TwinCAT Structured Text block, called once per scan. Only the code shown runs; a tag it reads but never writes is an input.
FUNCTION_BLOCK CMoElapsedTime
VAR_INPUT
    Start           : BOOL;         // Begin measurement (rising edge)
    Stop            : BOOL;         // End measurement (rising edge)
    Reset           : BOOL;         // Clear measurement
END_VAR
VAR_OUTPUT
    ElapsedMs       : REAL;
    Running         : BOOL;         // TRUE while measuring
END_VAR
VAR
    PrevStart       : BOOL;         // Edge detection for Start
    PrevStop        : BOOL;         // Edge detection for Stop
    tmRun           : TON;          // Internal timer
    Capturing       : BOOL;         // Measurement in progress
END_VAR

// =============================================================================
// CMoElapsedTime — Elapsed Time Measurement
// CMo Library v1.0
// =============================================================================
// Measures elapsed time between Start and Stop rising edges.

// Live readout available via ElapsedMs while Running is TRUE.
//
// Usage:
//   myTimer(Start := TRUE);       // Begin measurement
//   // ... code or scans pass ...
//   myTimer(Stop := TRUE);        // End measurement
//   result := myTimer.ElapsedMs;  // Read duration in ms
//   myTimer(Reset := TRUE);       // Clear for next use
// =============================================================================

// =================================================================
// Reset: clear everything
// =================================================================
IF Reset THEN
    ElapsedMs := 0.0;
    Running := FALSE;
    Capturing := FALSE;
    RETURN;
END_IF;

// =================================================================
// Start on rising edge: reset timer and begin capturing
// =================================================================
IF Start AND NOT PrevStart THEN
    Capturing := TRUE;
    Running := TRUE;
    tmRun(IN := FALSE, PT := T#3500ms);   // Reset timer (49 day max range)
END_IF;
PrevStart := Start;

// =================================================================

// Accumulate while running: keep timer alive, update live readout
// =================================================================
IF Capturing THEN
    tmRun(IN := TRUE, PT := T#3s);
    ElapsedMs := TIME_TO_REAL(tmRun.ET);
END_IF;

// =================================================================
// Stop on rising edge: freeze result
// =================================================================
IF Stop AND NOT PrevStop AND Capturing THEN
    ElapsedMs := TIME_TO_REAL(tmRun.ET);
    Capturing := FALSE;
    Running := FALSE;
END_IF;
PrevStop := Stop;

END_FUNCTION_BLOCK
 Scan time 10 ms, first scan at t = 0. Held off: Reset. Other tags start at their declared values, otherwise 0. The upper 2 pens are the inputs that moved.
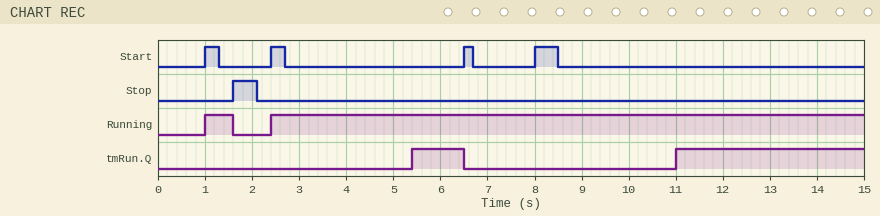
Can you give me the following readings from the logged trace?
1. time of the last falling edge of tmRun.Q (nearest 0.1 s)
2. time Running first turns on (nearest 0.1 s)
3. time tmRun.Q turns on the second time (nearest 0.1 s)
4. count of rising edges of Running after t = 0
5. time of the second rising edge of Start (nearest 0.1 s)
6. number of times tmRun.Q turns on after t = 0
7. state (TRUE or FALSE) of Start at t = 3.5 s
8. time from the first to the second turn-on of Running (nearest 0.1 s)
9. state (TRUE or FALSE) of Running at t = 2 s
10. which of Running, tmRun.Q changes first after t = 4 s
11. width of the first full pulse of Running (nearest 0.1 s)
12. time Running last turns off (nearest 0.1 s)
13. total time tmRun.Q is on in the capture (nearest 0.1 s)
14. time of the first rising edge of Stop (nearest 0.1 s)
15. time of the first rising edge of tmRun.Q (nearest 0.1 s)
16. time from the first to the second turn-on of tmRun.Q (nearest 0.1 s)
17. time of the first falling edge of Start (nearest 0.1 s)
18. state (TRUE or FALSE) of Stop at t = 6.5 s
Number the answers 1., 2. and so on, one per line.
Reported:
1. 6.5 s
2. 1.0 s
3. 11.0 s
4. 2
5. 2.4 s
6. 2
7. FALSE
8. 1.4 s
9. FALSE
10. tmRun.Q
11. 0.6 s
12. 1.6 s
13. 5.1 s
14. 1.6 s
15. 5.4 s
16. 5.6 s
17. 1.3 s
18. FALSE
